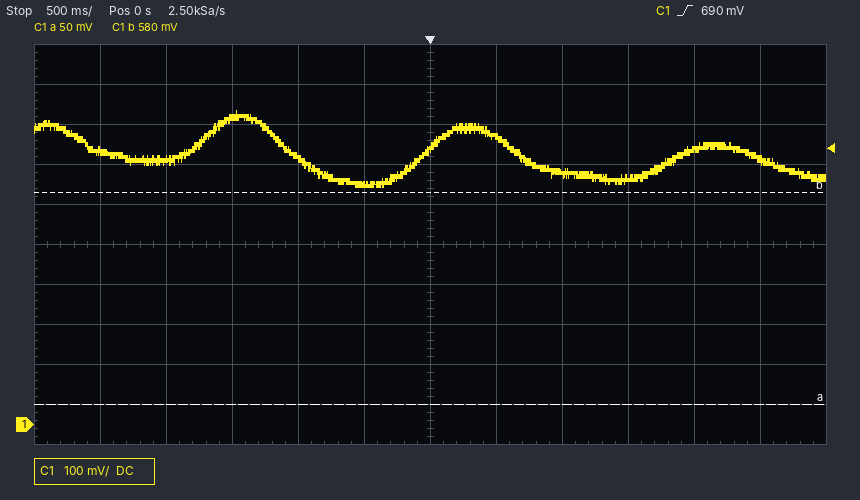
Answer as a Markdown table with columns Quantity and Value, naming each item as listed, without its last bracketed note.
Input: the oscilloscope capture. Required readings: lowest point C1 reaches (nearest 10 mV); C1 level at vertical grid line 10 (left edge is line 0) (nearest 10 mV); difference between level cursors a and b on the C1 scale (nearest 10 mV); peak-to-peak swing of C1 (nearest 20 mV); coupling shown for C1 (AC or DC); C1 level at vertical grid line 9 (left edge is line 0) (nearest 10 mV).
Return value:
| Quantity | Value |
|---|---|
| lowest point C1 reaches | 590 mV |
| C1 level at vertical grid line 10 (left edge is line 0) | 690 mV |
| difference between level cursors a and b on the C1 scale | 530 mV |
| peak-to-peak swing of C1 | 200 mV |
| coupling shown for C1 | DC |
| C1 level at vertical grid line 9 (left edge is line 0) | 620 mV |
